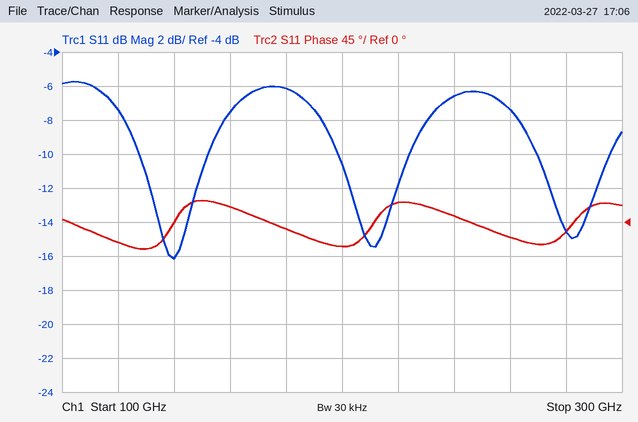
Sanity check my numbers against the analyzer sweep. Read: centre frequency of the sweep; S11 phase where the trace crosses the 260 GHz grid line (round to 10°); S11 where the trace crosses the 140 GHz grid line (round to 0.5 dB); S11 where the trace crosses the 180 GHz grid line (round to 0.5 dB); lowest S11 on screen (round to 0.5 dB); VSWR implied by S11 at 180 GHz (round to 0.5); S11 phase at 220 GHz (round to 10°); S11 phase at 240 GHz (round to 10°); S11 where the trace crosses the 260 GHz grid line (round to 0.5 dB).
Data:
200 GHz
-20°
-16.0 dB
-6.0 dB
-16.0 dB
3.0
30°
10°
-7.5 dB
